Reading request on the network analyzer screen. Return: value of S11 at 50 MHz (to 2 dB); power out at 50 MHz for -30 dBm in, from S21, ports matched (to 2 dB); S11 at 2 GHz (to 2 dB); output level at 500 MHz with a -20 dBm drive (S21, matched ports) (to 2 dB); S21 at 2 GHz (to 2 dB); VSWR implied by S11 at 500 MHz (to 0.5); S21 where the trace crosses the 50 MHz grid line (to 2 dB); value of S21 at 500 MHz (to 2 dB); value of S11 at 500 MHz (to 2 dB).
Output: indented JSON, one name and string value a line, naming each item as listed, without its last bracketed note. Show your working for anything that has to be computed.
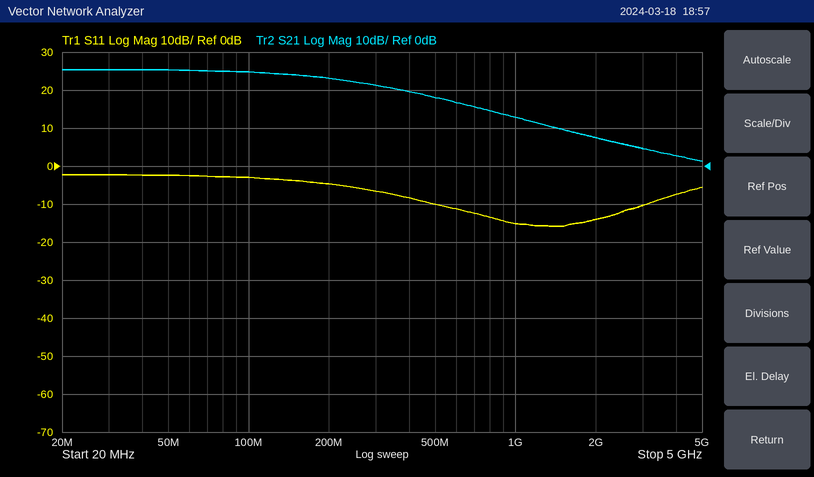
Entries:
{
  "value of S11 at 50 MHz": "-2 dB",
  "power out at 50 MHz for -30 dBm in, from S21, ports matched": "-30 dBm + (26 dB) = -4 dBm",
  "S11 at 2 GHz": "-14 dB",
  "output level at 500 MHz with a -20 dBm drive (S21, matched ports)": "-20 dBm + (18 dB) = -2 dBm",
  "S21 at 2 GHz": "8 dB",
  "VSWR implied by S11 at 500 MHz": "|Γ| = 10^(-10/20) = 0.3162; VSWR = (1 + 0.3162)/(1 − 0.3162) ≈ 1.92, so 2.0 to the nearest 0.5",
  "S21 where the trace crosses the 50 MHz grid line": "26 dB",
  "value of S21 at 500 MHz": "18 dB",
  "value of S11 at 500 MHz": "-10 dB"
}
